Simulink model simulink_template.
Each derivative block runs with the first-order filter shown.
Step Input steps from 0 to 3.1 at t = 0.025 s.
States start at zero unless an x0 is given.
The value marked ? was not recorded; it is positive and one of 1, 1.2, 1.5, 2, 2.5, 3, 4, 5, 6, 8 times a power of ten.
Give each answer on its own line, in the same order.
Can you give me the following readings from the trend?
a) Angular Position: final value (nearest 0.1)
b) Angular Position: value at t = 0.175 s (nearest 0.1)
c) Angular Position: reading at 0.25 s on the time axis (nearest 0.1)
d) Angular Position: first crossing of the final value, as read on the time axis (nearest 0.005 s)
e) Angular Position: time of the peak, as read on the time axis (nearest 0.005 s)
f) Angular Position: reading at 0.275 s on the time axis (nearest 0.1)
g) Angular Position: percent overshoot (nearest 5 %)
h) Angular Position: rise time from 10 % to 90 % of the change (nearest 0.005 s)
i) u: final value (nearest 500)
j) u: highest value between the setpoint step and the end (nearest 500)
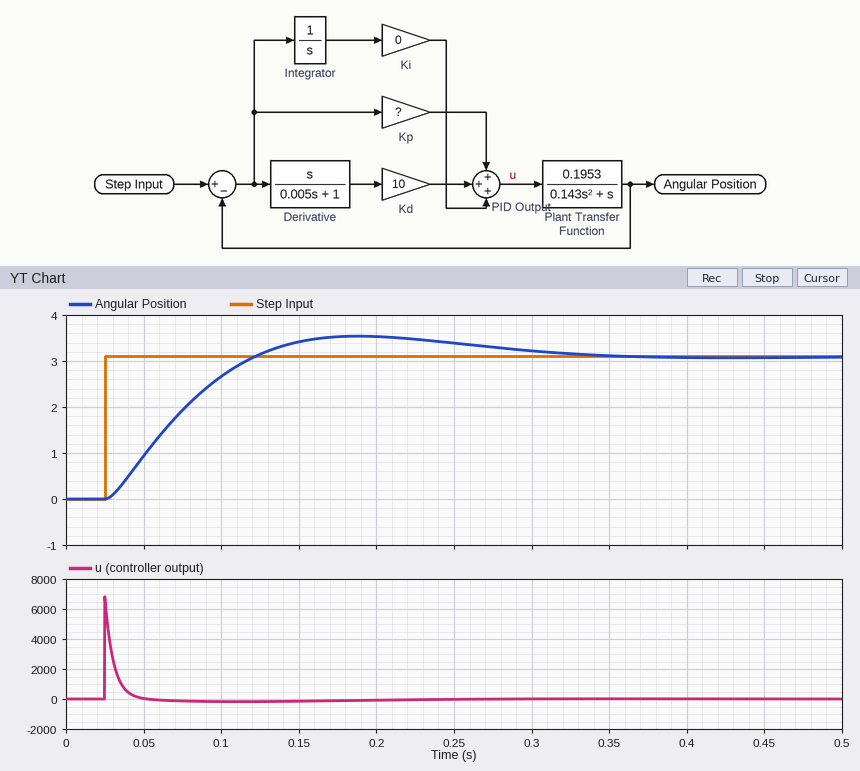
3.1
3.5
3.4
0.120 s
0.190 s
3.3
15 %
0.070 s
0
7000
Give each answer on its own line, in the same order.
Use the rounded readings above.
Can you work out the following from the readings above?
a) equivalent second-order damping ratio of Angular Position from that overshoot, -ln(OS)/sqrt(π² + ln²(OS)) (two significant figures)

0.52
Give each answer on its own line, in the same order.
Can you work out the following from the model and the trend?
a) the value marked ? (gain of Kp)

200
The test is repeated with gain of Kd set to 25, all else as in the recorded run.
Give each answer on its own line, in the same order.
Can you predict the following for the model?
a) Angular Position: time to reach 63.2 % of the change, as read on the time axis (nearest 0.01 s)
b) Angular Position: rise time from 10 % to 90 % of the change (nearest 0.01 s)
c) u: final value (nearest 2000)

0.05 s
0.05 s
0
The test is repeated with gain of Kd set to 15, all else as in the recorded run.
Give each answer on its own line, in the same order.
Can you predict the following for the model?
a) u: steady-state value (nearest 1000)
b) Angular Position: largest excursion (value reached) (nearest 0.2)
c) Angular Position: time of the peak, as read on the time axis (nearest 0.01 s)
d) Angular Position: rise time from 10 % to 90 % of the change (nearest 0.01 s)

0
3.4
0.18 s
0.06 s
